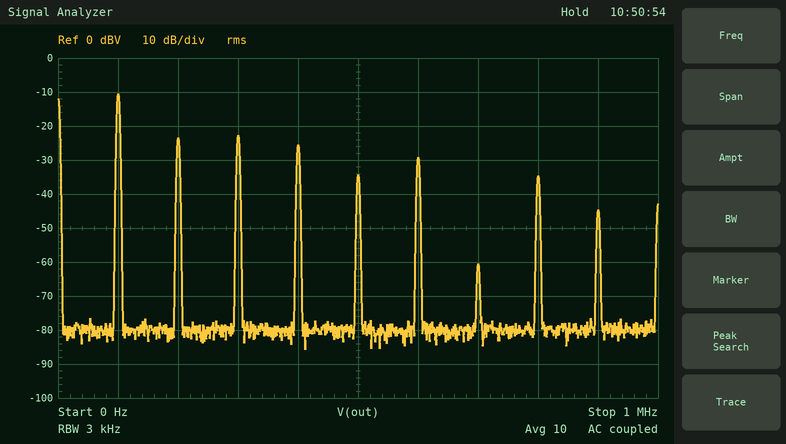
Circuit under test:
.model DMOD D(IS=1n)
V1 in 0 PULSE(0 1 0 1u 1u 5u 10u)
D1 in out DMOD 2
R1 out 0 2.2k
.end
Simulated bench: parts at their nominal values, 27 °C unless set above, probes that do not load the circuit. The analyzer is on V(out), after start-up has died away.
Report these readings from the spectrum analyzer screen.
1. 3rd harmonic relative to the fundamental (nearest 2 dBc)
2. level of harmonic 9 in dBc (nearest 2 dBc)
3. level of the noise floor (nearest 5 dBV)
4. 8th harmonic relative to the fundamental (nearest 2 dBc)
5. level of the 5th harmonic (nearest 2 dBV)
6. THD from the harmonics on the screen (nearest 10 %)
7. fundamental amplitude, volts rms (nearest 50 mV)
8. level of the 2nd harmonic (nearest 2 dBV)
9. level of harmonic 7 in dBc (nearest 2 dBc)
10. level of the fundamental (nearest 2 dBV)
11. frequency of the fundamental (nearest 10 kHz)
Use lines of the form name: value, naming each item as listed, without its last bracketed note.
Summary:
3rd harmonic relative to the fundamental: -12 dBc
level of harmonic 9 in dBc: -34 dBc
level of the noise floor: -80 dBV
8th harmonic relative to the fundamental: -24 dBc
level of the 5th harmonic: -34 dBV
THD from the harmonics on the screen: 40 %
fundamental amplitude, volts rms: 300 mV
level of the 2nd harmonic: -24 dBV
level of harmonic 7 in dBc: -50 dBc
level of the fundamental: -10 dBV
frequency of the fundamental: 100 kHz
